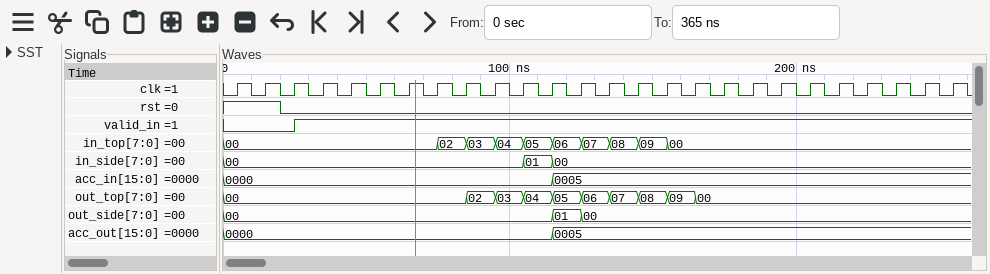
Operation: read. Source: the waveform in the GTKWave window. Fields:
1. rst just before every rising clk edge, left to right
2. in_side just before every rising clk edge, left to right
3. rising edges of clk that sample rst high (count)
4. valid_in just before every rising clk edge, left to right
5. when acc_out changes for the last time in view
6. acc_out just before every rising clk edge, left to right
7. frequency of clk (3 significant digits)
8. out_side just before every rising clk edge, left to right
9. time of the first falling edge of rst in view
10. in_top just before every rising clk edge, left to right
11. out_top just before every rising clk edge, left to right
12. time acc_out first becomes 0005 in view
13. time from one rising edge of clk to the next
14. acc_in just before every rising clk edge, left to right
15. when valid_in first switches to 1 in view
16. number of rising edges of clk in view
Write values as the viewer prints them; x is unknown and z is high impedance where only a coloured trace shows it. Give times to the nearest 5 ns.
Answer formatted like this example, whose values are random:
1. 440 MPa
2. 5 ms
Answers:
1. 1 1 0 0 0 0 0 0 0 0 0 0 0 0 0 0 0 0 0 0 0 0 0 0 0 0
2. 00, 00, 00, 00, 00, 00, 00, 00, 00, 00, 00, 01, 00, 00, 00, 00, 00, 00, 00, 00, 00, 00, 00, 00, 00, 00
3. 2
4. 0 0 0 1 1 1 1 1 1 1 1 1 1 1 1 1 1 1 1 1 1 1 1 1 1 1
5. 115 ns
6. 0000, 0000, 0000, 0000, 0000, 0000, 0000, 0000, 0000, 0000, 0000, 0000, 0005, 0005, 0005, 0005, 0005, 0005, 0005, 0005, 0005, 0005, 0005, 0005, 0005, 0005
7. 100 MHz
8. 00, 00, 00, 00, 00, 00, 00, 00, 00, 00, 00, 00, 01, 00, 00, 00, 00, 00, 00, 00, 00, 00, 00, 00, 00, 00
9. 20 ns
10. 00, 00, 00, 00, 00, 00, 00, 00, 02, 03, 04, 05, 06, 07, 08, 09, 00, 00, 00, 00, 00, 00, 00, 00, 00, 00
11. 00, 00, 00, 00, 00, 00, 00, 00, 00, 02, 03, 04, 05, 06, 07, 08, 09, 00, 00, 00, 00, 00, 00, 00, 00, 00
12. 115 ns
13. 10 ns
14. 0000, 0000, 0000, 0000, 0000, 0000, 0000, 0000, 0000, 0000, 0000, 0000, 0005, 0005, 0005, 0005, 0005, 0005, 0005, 0005, 0005, 0005, 0005, 0005, 0005, 0005
15. 25 ns
16. 26
